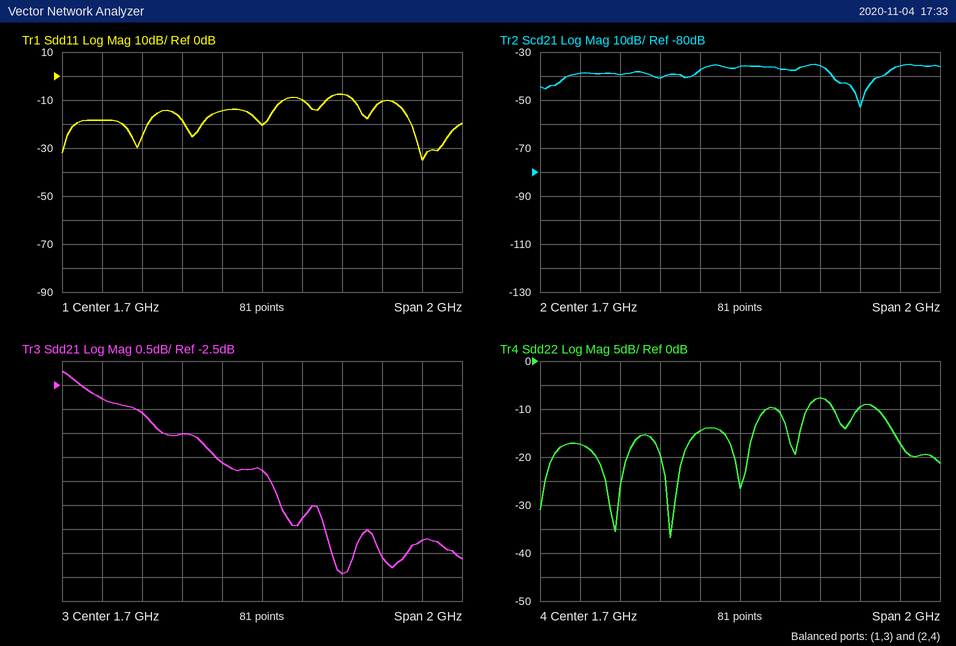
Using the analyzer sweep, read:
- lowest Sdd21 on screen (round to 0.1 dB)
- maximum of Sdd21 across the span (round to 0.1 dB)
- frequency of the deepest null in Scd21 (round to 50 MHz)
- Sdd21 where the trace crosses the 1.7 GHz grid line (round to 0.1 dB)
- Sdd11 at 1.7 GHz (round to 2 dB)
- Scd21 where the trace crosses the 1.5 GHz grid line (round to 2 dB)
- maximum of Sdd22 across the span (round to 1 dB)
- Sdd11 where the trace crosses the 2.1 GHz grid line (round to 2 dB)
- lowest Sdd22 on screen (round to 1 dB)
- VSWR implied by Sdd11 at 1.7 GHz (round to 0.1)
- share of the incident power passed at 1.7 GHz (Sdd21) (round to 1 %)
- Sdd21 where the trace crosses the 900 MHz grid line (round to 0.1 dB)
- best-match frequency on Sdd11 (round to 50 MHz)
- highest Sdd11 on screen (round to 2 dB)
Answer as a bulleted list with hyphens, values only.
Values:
- -6.4 dB
- -2.2 dB
- 2.30 GHz
- -4.3 dB
- -20 dB
- -38 dB
- -8 dB
- -8 dB
- -37 dB
- 1.2
- 37 %
- -2.8 dB
- 2.50 GHz
- -8 dB
